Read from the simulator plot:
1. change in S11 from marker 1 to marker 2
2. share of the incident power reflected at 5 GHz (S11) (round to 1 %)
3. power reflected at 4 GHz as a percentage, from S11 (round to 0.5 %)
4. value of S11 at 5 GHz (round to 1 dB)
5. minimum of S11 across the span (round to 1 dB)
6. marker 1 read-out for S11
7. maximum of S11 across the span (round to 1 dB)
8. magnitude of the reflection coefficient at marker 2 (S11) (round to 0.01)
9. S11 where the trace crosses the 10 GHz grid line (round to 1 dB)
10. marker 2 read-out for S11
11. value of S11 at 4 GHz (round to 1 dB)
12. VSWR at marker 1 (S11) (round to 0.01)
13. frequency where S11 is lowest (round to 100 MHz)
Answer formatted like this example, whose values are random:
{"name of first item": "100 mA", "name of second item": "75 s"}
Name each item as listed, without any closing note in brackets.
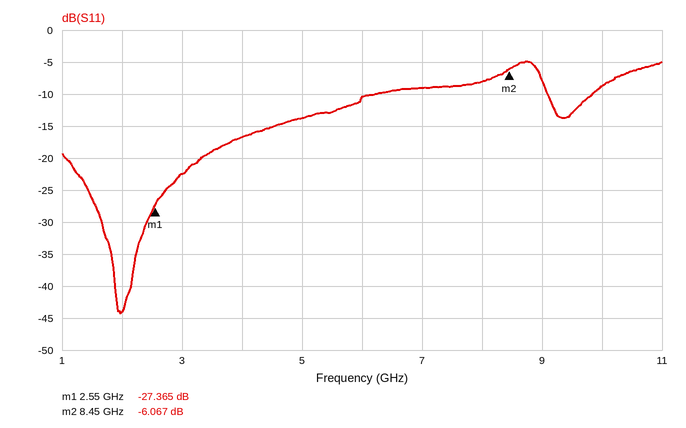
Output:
{"change in S11 from marker 1 to marker 2": "21.298 dB", "share of the incident power reflected at 5 GHz (S11)": "4 %", "power reflected at 4 GHz as a percentage, from S11": "2.0 %", "value of S11 at 5 GHz": "-14 dB", "minimum of S11 across the span": "-44 dB", "marker 1 read-out for S11": "-27.365 dB", "maximum of S11 across the span": "-5 dB", "magnitude of the reflection coefficient at marker 2 (S11)": "0.50", "S11 where the trace crosses the 10 GHz grid line": "-9 dB", "marker 2 read-out for S11": "-6.067 dB", "value of S11 at 4 GHz": "-17 dB", "VSWR at marker 1 (S11)": "1.09", "frequency where S11 is lowest": "2.0 GHz"}
